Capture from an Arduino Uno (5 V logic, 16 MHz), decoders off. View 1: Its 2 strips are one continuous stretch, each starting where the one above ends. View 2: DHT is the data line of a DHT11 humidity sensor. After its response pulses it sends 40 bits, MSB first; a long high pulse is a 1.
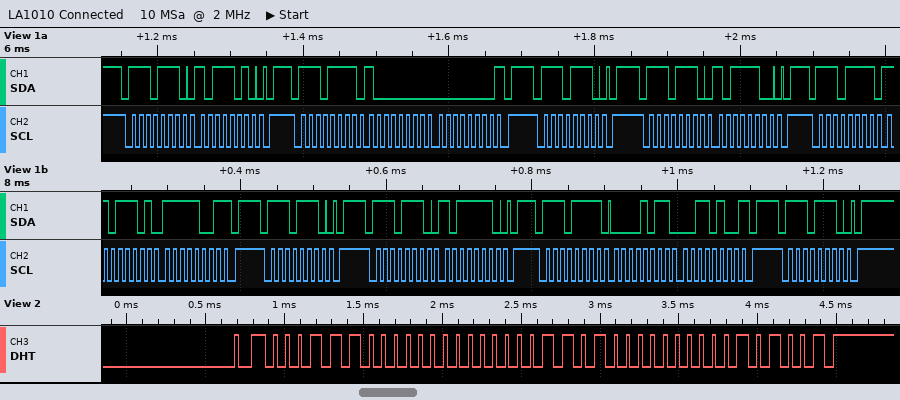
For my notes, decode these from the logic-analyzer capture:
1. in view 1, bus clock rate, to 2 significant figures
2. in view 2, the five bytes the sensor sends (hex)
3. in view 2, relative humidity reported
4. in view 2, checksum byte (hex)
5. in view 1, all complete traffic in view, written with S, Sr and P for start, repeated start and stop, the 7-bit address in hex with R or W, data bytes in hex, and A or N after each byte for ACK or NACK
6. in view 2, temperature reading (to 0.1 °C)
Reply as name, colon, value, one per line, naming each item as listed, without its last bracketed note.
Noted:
in view 1, bus clock rate, to 2 significant figures: 100 kHz
in view 2, the five bytes the sensor sends: 1C 00 0D 00 29
in view 2, relative humidity reported: 28 %
in view 2, checksum byte: 0x29
in view 1, all complete traffic in view, written with S, Sr and P for start, repeated start and stop, the 7-bit address in hex with R or W, data bytes in hex, and A or N after each byte for ACK or NACK: S 77W A BA A P S 77R A 80 A 00 N P S 77W A P S 77W A BC A P S 77R A DD A F9 N P S 77W A P S 77W A BE A P S 77R A 0B A 34 N P S 77W A P
in view 2, temperature reading: 13.0 °C
